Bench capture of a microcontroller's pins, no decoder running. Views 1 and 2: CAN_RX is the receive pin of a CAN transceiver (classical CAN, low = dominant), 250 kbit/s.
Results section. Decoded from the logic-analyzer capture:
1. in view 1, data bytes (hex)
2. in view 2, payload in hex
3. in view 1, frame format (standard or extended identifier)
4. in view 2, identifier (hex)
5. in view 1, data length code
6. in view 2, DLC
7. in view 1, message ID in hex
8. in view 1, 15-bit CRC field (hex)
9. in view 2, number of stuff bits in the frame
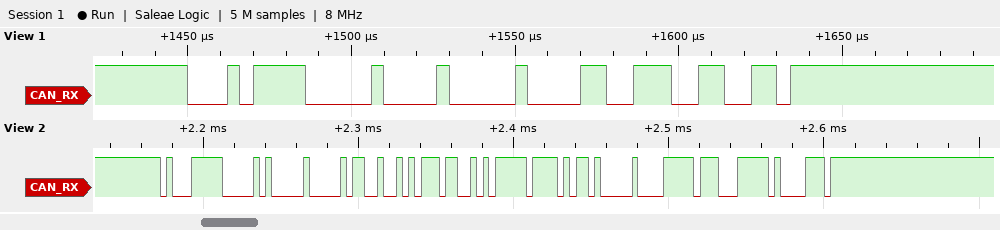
00
00 C9 5D 95 FF 5A 00 FF
standard
0x47C
1
8
0x178
0x3399
8
